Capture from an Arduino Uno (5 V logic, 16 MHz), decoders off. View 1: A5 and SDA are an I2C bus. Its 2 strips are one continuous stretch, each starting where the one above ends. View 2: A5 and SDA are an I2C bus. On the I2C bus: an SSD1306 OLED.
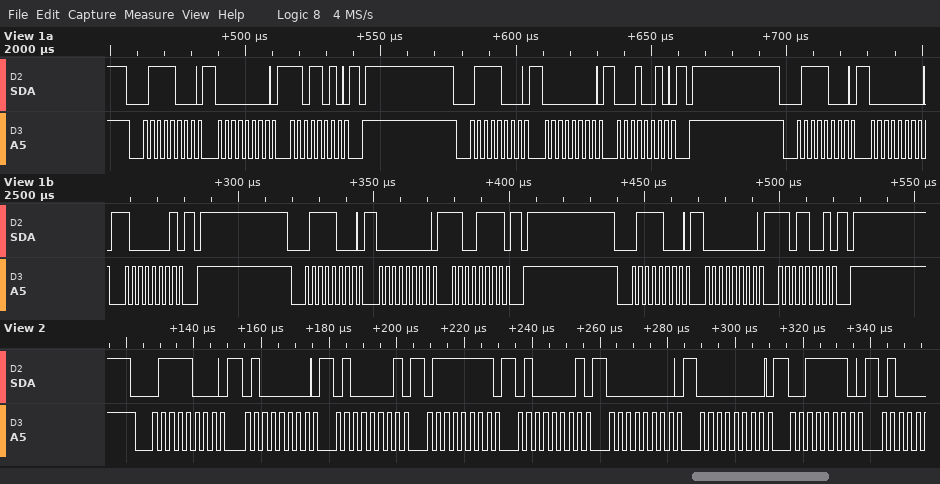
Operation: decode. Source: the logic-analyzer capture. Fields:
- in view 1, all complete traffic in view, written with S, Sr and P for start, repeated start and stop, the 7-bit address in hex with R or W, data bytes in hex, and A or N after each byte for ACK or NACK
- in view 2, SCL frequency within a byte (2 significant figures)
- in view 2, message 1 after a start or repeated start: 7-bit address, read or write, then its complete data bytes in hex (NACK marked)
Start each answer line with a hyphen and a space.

- S 3CW A 00 A DA A P S 3CW A 00 A 12 A P S 3CW A 00 A 81 A P S 3CW A 00 A CF A P S 3CW A 00 A D9 A P
- 400 kHz
- 0x3C write: 40 41 7F 41 00 00 3E
